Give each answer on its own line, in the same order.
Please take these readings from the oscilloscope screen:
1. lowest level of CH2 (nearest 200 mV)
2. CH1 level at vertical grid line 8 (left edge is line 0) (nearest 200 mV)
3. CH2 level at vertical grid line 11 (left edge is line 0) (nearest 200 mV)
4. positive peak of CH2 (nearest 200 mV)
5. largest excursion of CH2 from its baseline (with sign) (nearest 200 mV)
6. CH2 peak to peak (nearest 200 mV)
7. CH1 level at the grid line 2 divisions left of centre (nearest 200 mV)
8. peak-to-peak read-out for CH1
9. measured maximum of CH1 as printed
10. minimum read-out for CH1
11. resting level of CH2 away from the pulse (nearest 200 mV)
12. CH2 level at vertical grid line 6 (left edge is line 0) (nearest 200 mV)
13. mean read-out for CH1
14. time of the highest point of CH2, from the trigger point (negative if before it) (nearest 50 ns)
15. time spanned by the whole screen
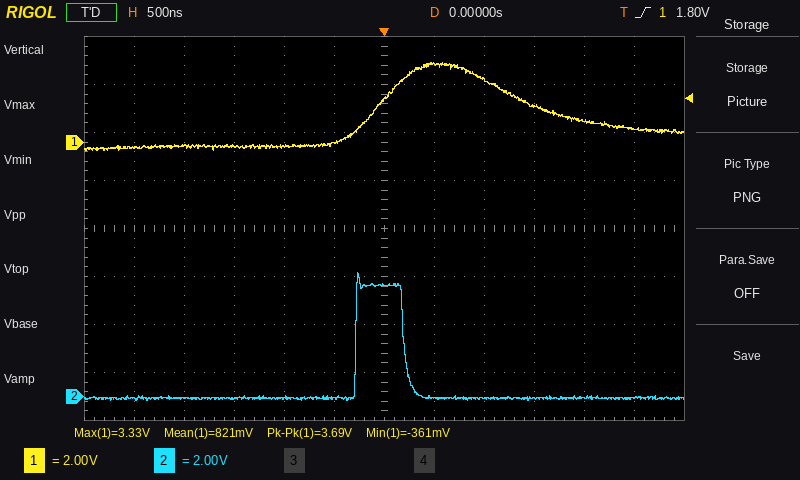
-200 mV
2.6 V
0.0 V
5.2 V
+5.2 V
5.4 V
-200 mV
3.69 V
3.33 V
-361 mV
0.0 V
4.6 V
821 mV
-250 ns
6 µs
